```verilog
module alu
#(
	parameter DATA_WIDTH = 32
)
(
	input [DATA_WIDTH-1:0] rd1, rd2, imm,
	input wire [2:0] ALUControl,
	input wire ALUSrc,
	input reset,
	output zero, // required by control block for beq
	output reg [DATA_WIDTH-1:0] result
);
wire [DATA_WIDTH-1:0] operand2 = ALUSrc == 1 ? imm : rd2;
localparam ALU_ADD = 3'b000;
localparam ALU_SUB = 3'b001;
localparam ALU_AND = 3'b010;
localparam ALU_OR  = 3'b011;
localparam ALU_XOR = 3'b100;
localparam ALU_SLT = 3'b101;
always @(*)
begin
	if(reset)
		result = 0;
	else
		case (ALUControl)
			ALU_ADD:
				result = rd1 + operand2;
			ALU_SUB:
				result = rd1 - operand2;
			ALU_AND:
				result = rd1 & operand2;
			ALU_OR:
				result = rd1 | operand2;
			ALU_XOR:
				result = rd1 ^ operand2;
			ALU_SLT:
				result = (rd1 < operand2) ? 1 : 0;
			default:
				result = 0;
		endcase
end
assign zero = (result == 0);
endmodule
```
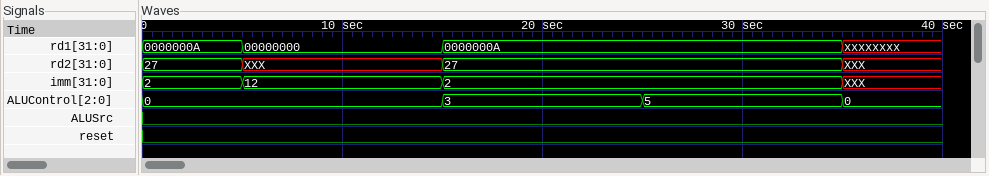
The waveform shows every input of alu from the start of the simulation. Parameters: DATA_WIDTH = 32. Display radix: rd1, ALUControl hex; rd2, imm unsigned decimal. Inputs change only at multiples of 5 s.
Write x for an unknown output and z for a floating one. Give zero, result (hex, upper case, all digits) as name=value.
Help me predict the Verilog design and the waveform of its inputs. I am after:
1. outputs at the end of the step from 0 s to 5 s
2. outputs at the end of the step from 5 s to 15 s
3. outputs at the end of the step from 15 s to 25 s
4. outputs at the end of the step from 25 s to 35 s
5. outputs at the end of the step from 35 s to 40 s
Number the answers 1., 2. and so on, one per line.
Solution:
1. zero=0, result=00000025
2. zero=x, result=x
3. zero=0, result=0000001B
4. zero=0, result=00000001
5. zero=x, result=x
